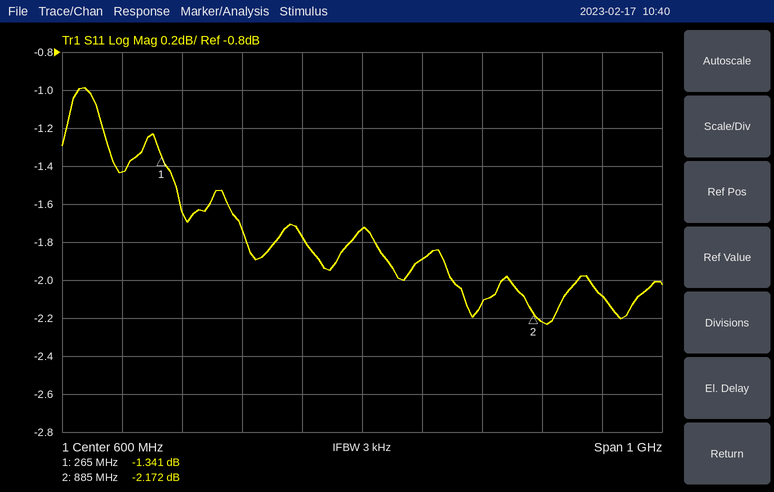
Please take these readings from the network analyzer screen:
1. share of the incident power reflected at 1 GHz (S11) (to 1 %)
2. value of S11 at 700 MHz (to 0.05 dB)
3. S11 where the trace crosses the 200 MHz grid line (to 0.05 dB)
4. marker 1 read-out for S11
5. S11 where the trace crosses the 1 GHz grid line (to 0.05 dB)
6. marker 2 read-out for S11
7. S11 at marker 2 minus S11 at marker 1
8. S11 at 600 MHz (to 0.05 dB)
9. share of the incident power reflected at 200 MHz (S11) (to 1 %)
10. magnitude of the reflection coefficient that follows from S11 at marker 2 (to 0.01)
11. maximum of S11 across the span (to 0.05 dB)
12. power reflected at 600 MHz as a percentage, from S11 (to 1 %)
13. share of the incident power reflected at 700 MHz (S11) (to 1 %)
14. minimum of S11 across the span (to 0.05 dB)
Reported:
62 %
-1.90 dB
-1.45 dB
-1.341 dB
-2.10 dB
-2.172 dB
-0.831 dB
-1.75 dB
72 %
0.78
-1.00 dB
67 %
65 %
-2.25 dB
